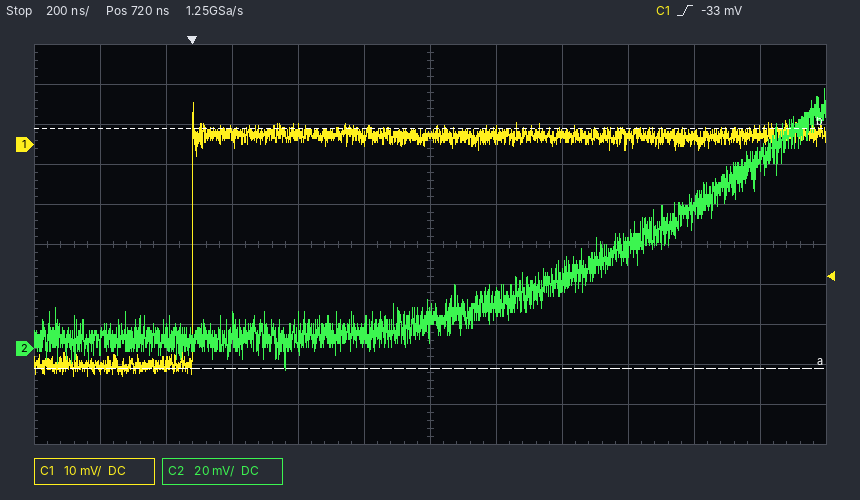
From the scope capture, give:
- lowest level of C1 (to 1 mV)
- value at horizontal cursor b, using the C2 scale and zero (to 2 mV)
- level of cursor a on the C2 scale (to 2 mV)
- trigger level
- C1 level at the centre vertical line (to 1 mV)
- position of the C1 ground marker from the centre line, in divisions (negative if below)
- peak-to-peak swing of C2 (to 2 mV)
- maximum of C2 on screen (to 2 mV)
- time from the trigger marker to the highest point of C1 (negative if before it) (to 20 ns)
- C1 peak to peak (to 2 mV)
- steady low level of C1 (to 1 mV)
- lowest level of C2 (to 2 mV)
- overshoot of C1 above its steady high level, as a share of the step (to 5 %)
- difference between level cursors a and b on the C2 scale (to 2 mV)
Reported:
-58 mV
110 mV
-10 mV
-33 mV
2 mV
+2.5 div
140 mV
130 mV
0 ns
68 mV
-55 mV
-10 mV
15 %
120 mV
